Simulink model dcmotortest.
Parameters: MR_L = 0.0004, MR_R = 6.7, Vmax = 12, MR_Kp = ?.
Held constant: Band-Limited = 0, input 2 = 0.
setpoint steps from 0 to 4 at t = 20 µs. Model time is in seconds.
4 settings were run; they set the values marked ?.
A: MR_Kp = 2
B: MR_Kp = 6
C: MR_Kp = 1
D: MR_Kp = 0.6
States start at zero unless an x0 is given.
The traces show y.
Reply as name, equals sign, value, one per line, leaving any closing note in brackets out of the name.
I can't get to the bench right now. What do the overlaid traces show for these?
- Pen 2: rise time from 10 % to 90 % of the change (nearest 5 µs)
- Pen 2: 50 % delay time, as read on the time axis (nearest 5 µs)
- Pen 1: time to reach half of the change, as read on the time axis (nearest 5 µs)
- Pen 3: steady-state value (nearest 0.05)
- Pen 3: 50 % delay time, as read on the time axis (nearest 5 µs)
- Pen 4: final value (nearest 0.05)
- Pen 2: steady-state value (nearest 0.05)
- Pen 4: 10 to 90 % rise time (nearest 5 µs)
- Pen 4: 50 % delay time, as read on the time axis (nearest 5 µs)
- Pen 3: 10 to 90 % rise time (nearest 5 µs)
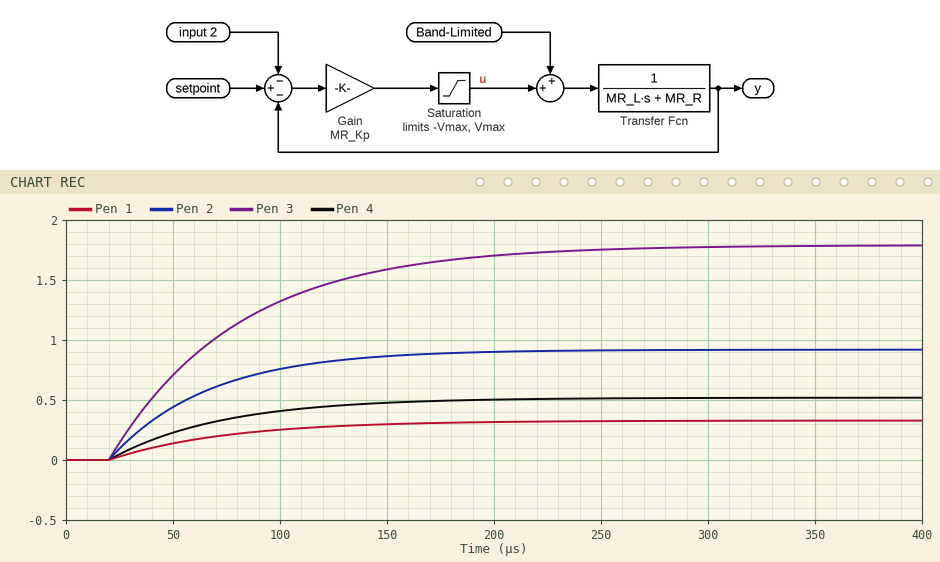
Pen 2: rise time from 10 % to 90 % of the change = 100 µs
Pen 2: 50 % delay time, as read on the time axis = 50 µs
Pen 1: time to reach half of the change, as read on the time axis = 60 µs
Pen 3: steady-state value = 1.80
Pen 3: 50 % delay time, as read on the time axis = 60 µs
Pen 4: final value = 0.50
Pen 2: steady-state value = 0.90
Pen 4: 10 to 90 % rise time = 115 µs
Pen 4: 50 % delay time, as read on the time axis = 55 µs
Pen 3: 10 to 90 % rise time = 130 µs
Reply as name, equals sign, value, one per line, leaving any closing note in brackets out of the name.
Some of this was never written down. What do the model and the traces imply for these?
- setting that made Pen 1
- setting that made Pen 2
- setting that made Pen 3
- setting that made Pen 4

setting that made Pen 1 = D
setting that made Pen 2 = A
setting that made Pen 3 = B
setting that made Pen 4 = C
